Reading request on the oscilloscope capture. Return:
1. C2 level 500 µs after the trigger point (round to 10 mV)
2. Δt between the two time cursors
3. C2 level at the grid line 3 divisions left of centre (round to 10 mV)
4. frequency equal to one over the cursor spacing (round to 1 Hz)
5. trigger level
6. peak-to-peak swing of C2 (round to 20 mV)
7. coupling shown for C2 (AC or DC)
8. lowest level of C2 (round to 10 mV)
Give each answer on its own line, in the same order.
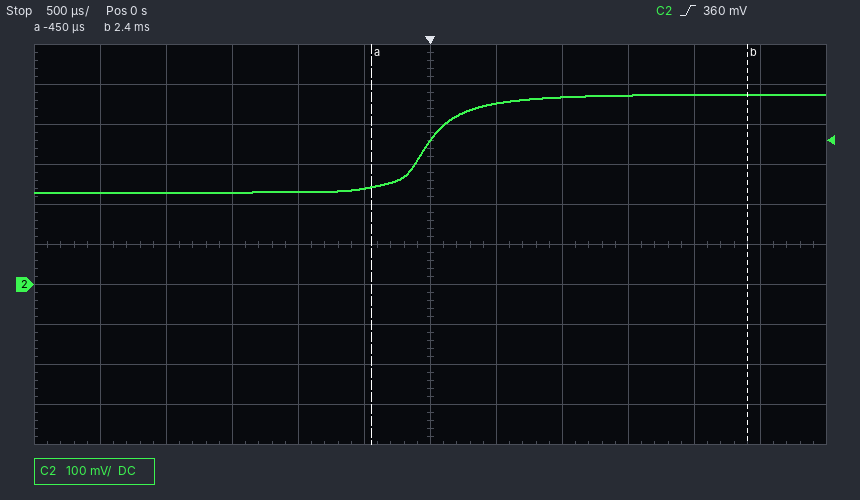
450 mV
2.85 ms
230 mV
351 Hz
360 mV
240 mV
DC
230 mV
